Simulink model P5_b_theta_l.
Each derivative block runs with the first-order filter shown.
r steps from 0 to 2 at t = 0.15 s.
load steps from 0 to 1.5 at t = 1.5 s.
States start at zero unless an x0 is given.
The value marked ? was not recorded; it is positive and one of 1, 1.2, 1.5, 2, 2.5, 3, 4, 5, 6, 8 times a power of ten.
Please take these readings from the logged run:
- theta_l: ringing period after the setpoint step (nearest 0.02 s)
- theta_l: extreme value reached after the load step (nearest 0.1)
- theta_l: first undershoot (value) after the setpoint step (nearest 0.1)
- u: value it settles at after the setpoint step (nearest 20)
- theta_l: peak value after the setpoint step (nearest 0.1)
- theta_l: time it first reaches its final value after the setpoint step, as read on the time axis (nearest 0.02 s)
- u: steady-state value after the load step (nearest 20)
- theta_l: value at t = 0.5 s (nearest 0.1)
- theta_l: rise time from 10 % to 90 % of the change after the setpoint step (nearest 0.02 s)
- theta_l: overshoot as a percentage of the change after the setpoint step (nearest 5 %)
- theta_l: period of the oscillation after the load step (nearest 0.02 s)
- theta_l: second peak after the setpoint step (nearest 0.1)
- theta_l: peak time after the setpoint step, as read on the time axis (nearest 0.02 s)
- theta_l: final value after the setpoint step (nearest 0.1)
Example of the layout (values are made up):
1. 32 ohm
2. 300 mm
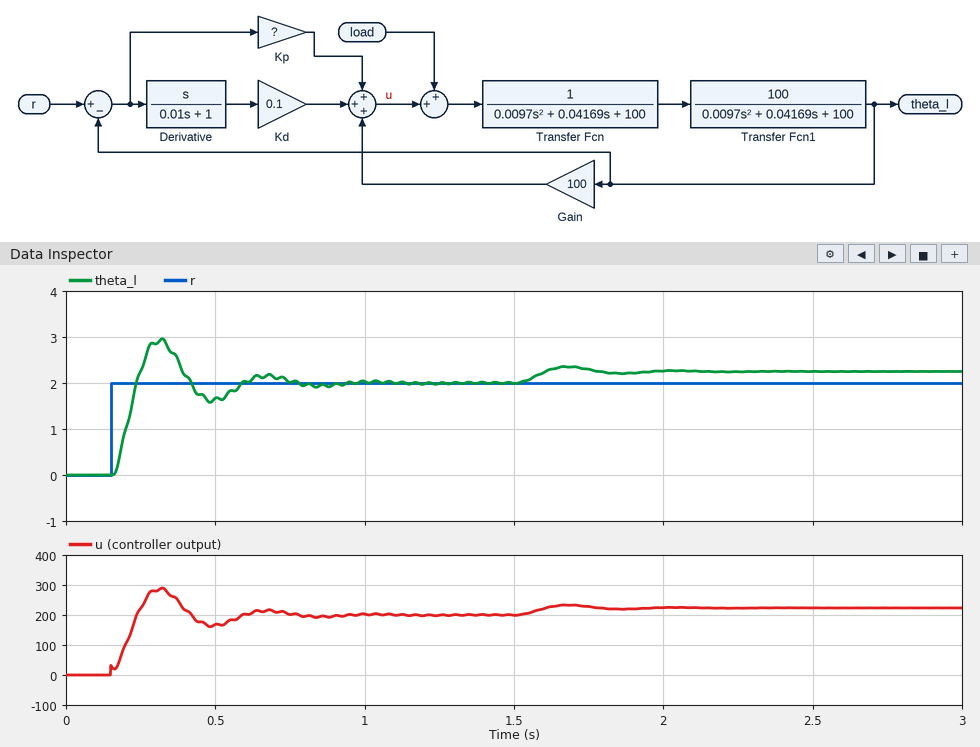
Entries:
1. 0.36 s
2. 2.4
3. 1.6
4. 200
5. 3.0
6. 0.24 s
7. 220
8. 1.7
9. 0.06 s
10. 50 %
11. 0.36 s
12. 2.2
13. 0.32 s
14. 2.0
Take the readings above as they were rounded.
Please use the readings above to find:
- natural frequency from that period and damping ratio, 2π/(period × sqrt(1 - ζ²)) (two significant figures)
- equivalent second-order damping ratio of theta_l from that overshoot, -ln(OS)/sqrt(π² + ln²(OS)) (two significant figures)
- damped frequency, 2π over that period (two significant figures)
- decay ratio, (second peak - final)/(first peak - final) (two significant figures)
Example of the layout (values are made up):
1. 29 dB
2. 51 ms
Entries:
1. 18 rad/s
2. 0.22
3. 17 rad/s
4. 0.20
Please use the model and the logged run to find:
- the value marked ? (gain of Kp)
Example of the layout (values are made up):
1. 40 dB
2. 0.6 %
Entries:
1. 6
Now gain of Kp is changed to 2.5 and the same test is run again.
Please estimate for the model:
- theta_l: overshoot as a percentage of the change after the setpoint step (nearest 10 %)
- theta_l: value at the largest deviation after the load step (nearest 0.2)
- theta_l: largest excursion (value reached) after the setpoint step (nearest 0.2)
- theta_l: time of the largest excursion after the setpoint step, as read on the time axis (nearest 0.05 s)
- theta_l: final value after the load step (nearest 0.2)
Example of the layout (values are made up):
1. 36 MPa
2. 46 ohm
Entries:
1. 30 %
2. 2.8
3. 2.6
4. 0.40 s
5. 2.6
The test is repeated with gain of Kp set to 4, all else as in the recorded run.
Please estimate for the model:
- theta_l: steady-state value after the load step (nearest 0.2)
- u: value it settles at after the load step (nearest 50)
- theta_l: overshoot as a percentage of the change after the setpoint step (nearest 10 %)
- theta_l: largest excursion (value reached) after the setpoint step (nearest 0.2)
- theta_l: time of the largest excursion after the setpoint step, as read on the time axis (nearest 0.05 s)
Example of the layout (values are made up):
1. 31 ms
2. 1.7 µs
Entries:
1. 2.4
2. 250
3. 40 %
4. 2.8
5. 0.35 s
